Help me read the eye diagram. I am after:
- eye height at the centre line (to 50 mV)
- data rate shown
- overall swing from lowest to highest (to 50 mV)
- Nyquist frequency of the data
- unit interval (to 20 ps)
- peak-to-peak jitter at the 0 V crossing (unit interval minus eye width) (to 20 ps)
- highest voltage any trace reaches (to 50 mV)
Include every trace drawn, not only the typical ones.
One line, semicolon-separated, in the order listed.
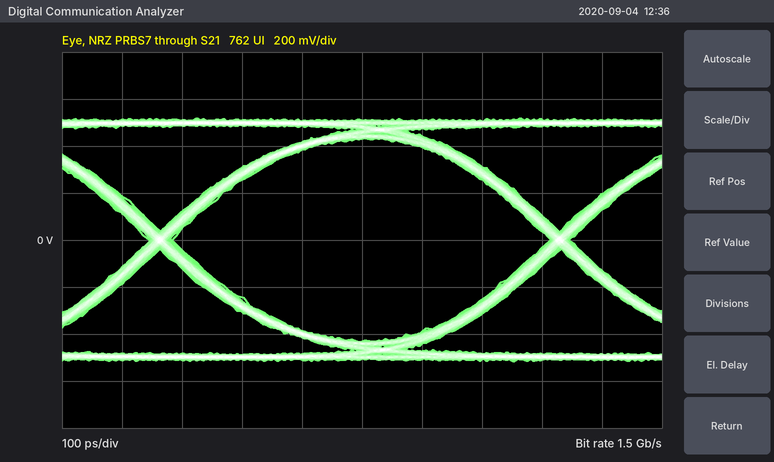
850 mV; 1.5 Gb/s; 1.05 V; 750 MHz; 660 ps; 40 ps; 500 mV
